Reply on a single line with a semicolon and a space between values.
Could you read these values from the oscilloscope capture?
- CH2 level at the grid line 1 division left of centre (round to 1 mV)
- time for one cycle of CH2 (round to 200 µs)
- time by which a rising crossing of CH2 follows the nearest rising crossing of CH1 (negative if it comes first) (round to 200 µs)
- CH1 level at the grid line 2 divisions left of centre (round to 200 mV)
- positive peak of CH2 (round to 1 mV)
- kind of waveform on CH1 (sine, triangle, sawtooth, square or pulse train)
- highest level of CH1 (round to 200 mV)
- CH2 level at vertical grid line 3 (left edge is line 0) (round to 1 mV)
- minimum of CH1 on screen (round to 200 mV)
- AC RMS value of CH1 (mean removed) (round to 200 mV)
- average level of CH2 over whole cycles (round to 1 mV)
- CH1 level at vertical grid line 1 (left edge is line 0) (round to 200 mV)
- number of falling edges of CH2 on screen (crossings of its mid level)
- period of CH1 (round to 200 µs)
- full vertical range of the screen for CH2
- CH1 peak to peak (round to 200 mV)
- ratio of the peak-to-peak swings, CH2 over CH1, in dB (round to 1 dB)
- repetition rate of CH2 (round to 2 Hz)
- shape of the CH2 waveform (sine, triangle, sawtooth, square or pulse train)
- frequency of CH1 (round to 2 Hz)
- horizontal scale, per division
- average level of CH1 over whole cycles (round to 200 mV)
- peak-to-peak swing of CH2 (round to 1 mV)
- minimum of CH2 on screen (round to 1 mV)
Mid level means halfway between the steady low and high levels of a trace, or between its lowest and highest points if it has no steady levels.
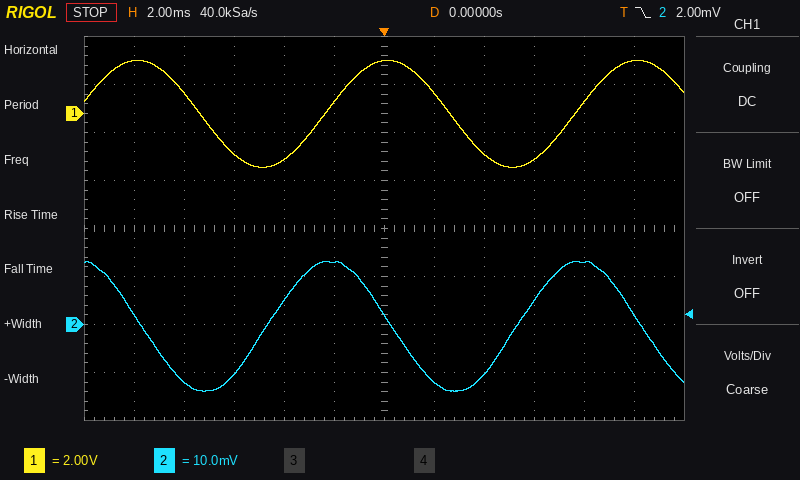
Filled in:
13 mV; 10.0 ms; -2.4 ms; -2.0 V; 13 mV; sine; 2.2 V; -10 mV; -2.2 V; 1.6 V; 0 mV; 2.2 V; 3; 10.0 ms; 80 mV; 4.4 V; -44 dB; 100 Hz; sine; 100 Hz; 2 ms; 0.0 V; 27 mV; -14 mV
